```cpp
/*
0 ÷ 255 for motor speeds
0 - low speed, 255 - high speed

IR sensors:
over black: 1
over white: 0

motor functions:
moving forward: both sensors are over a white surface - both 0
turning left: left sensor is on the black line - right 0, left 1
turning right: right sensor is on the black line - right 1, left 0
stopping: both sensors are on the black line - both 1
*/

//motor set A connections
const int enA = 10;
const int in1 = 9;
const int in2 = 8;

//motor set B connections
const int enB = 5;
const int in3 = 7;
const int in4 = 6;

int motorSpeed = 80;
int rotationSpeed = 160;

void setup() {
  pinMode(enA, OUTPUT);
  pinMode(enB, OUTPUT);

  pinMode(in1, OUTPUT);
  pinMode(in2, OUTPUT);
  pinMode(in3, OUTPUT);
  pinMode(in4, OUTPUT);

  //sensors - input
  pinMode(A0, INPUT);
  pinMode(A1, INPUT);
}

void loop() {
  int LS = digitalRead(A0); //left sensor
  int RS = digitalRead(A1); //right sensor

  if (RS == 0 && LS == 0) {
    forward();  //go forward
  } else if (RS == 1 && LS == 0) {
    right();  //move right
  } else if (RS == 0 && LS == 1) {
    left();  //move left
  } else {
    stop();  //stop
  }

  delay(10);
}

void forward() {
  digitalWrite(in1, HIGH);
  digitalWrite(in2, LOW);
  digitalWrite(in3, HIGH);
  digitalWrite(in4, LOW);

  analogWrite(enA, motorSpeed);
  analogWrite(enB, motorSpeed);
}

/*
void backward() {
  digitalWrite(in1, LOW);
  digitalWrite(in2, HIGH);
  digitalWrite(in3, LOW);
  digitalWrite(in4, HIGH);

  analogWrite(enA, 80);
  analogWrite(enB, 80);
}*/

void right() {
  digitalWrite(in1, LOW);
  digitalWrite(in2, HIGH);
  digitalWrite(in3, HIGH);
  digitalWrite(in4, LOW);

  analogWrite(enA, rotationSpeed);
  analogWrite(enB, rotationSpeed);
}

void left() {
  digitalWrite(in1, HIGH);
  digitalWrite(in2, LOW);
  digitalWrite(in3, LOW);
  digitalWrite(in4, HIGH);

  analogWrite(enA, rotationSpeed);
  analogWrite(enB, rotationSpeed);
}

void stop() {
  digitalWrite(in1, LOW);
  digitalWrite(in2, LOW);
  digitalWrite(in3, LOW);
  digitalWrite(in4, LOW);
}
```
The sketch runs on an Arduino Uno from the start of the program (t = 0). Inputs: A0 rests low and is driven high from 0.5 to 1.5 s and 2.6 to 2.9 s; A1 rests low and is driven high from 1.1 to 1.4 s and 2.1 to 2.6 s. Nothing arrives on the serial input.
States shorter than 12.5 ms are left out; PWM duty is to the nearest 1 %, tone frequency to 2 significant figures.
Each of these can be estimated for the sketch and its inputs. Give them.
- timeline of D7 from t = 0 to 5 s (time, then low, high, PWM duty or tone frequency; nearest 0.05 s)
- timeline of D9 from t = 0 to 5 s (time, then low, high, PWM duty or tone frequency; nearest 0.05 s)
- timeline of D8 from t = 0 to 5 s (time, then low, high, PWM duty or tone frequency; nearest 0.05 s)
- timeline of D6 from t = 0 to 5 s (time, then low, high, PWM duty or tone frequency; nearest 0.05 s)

0 s high; 0.5 s low; 1.5 s high; 2.6 s low; 2.9 s high
0 s high; 1.1 s low; 1.4 s high; 2.1 s low; 2.6 s high
0 s low; 2.1 s high; 2.6 s low
0 s low; 0.5 s high; 1.1 s low; 1.4 s high; 1.5 s low; 2.6 s high; 2.9 s low
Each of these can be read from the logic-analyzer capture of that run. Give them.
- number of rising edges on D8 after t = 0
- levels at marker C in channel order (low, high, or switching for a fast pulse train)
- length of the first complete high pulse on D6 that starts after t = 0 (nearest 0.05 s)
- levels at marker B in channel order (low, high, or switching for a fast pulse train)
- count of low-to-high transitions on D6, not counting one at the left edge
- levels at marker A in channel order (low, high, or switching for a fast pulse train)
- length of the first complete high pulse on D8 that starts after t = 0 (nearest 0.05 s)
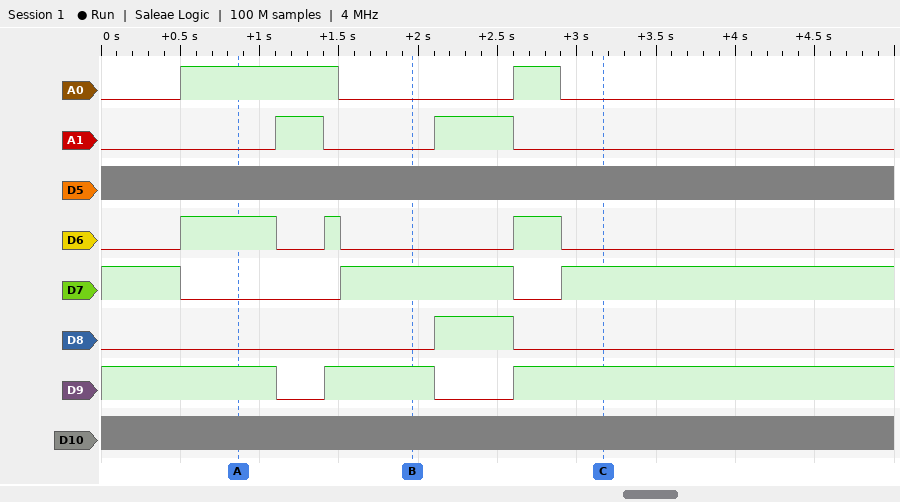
1
A0 low, A1 low, D5 switching, D6 low, D7 high, D8 low, D9 high, D10 switching
0.60 s
A0 low, A1 low, D5 switching, D6 low, D7 high, D8 low, D9 high, D10 switching
3
A0 high, A1 low, D5 switching, D6 high, D7 low, D8 low, D9 high, D10 switching
0.50 s
